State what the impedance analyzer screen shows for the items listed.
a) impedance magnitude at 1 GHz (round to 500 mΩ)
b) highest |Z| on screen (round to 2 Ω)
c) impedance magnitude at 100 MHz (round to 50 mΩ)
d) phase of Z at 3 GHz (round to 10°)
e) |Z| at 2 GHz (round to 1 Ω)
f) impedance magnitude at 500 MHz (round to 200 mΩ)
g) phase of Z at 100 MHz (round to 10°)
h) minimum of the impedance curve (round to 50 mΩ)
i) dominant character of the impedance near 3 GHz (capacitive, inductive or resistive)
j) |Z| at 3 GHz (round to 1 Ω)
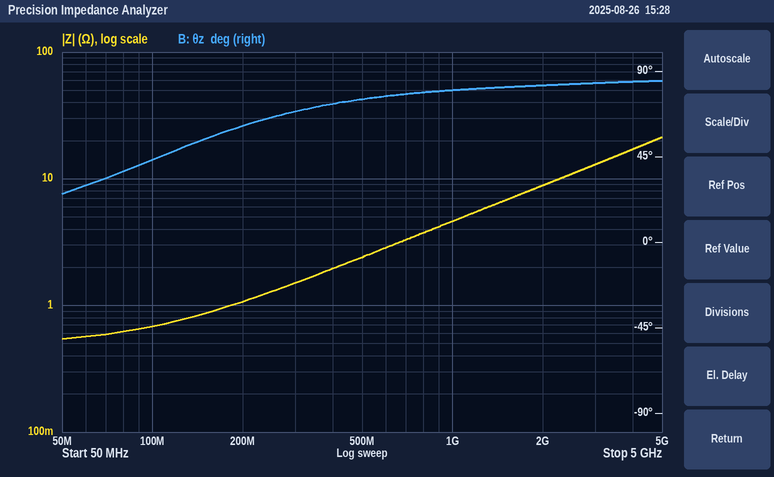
4.5 Ω
22 Ω
700 mΩ
80°
9 Ω
2.4 Ω
40°
550 mΩ
inductive
13 Ω
